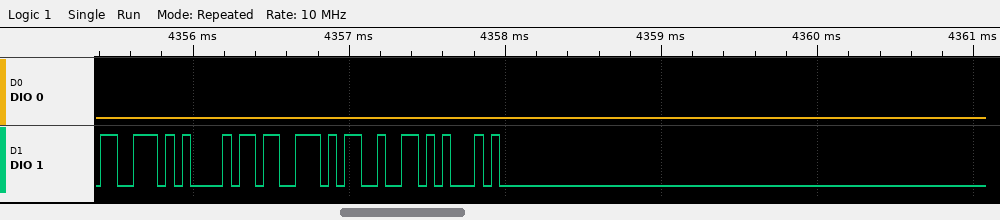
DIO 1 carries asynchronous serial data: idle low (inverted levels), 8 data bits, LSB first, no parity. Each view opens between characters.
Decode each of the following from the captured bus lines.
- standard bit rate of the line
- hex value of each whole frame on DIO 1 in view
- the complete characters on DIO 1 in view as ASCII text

19200 baud
46, 2F, 46, 36, 5D
"F/F6]"
